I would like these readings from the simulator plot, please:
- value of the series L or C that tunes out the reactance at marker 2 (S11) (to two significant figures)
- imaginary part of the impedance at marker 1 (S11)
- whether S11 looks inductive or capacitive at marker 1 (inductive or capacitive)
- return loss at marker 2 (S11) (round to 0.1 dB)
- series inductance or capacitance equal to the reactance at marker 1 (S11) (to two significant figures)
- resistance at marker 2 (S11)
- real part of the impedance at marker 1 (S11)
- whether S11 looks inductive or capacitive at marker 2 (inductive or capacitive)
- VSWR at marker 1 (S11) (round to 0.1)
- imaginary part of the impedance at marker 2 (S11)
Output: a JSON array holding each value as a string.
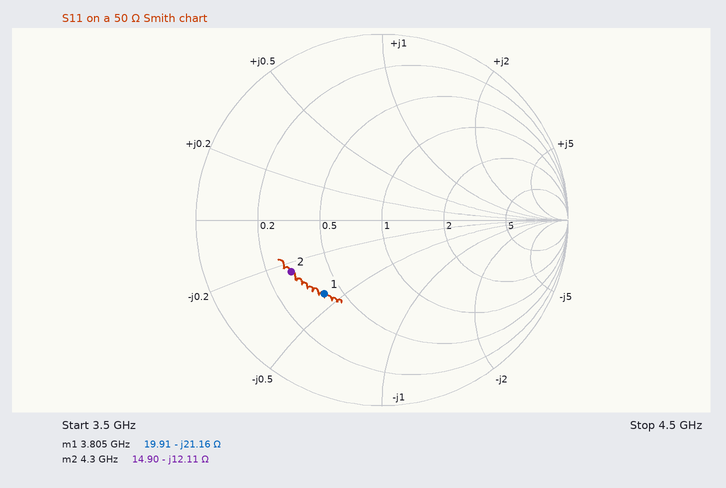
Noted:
["450 pH", "-21.16 Ω", "capacitive", "5.0 dB", "2.0 pF", "14.90 Ω", "19.91 Ω", "capacitive", "3.0", "-12.11 Ω"]
